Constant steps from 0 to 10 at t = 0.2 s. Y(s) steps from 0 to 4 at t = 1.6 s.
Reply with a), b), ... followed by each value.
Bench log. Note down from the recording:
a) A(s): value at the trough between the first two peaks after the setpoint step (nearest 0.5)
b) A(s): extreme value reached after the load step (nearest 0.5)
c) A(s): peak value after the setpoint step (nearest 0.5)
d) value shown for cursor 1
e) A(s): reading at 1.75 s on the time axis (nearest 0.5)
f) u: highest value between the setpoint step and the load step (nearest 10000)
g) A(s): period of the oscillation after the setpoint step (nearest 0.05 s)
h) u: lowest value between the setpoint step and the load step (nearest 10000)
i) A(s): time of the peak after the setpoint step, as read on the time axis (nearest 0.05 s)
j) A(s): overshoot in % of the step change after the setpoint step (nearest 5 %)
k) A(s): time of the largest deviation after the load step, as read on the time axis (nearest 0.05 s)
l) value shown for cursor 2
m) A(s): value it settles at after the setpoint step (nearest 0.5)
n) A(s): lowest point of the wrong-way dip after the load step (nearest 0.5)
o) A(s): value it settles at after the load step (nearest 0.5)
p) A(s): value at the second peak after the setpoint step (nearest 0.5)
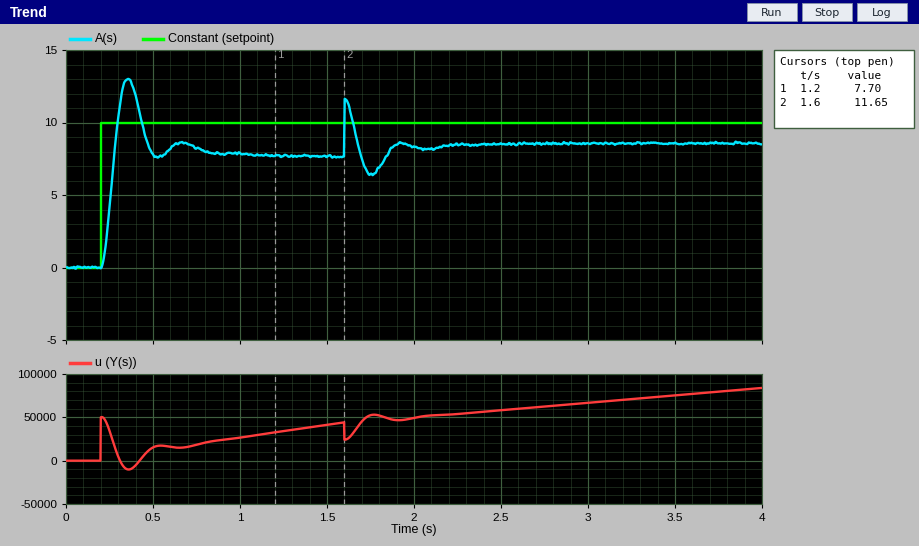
a) 7.5
b) 11.5
c) 13.0
d) 7.70
e) 6.5
f) 50000
g) 0.30 s
h) -10000
i) 0.35 s
j) 70 %
k) 1.60 s
l) 11.65
m) 7.5
n) 6.5
o) 8.5
p) 8.5
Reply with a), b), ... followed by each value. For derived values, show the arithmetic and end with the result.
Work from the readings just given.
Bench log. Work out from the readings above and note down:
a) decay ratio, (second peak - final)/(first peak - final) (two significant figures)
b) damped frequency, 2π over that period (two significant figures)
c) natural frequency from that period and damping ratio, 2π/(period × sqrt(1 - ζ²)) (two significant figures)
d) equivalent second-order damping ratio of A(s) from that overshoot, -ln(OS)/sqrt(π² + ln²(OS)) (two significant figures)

a) (8.5 - 7.5) / (13 - 7.5) = 0.18
b) 2π / 0.3 = 21 rad/s
c) 2π / (0.3 × sqrt(1 - 0.11²)) = 21 rad/s
d) ln(0.7) = -0.357; 0.357 / sqrt(9.870 + 0.127) = 0.11
